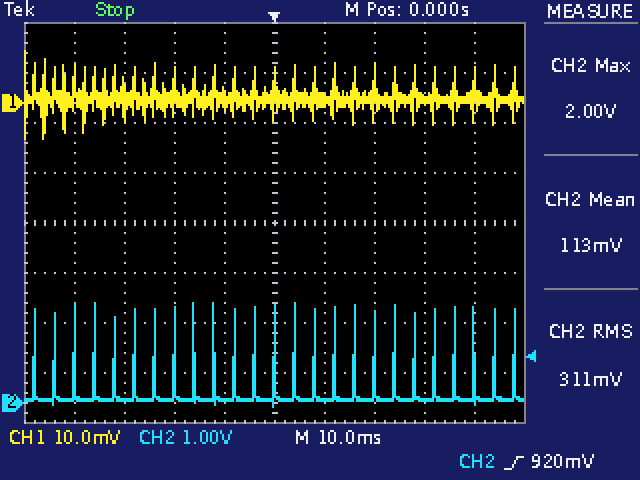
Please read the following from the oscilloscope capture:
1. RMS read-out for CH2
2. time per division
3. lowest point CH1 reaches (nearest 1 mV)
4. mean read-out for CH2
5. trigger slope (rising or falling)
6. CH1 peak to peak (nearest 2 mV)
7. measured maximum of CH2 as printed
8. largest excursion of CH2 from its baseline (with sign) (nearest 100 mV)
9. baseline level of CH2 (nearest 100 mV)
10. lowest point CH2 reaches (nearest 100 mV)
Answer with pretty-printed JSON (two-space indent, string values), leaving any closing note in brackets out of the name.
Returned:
{
  "RMS read-out for CH2": "311 mV",
  "time per division": "10 ms",
  "lowest point CH1 reaches": "-7 mV",
  "mean read-out for CH2": "113 mV",
  "trigger slope": "rising",
  "CH1 peak to peak": "18 mV",
  "measured maximum of CH2 as printed": "2.00 V",
  "largest excursion of CH2 from its baseline (with sign)": "+1.9 V",
  "baseline level of CH2": "100 mV",
  "lowest point CH2 reaches": "-100 mV"
}
